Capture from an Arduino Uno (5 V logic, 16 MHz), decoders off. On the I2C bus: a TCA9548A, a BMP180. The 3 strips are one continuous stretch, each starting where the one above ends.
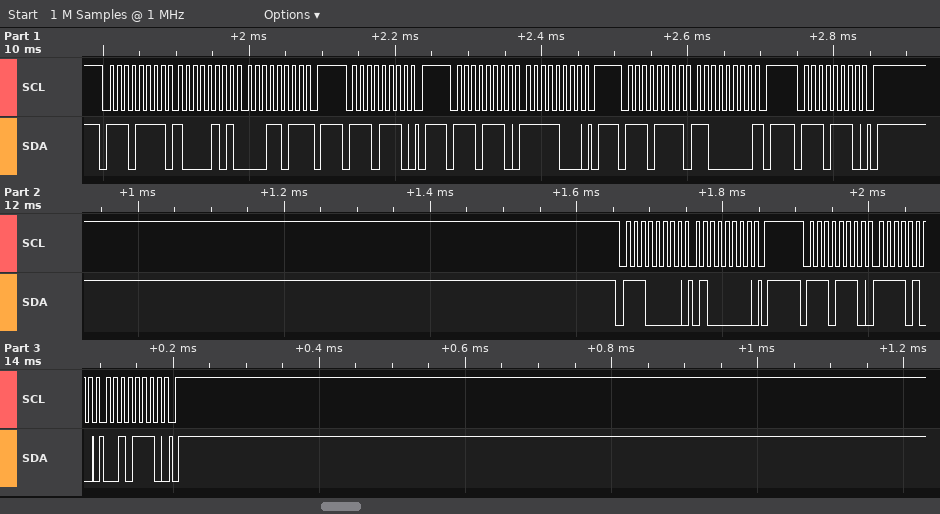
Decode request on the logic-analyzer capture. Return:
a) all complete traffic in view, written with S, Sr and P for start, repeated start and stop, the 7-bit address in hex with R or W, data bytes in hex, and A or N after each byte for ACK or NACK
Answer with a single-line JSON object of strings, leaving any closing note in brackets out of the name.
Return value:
{"all complete traffic in view, written with S, Sr and P for start, repeated start and stop, the 7-bit address in hex with R or W, data bytes in hex, and A or N after each byte for ACK or NACK": "S 77R A 85 A 1B N P S 77W A P S 77W A F8 A P S 77R A C0 N P S 77W A P S 70W A 40 A P S 77W A F4 A 2E A P"}
